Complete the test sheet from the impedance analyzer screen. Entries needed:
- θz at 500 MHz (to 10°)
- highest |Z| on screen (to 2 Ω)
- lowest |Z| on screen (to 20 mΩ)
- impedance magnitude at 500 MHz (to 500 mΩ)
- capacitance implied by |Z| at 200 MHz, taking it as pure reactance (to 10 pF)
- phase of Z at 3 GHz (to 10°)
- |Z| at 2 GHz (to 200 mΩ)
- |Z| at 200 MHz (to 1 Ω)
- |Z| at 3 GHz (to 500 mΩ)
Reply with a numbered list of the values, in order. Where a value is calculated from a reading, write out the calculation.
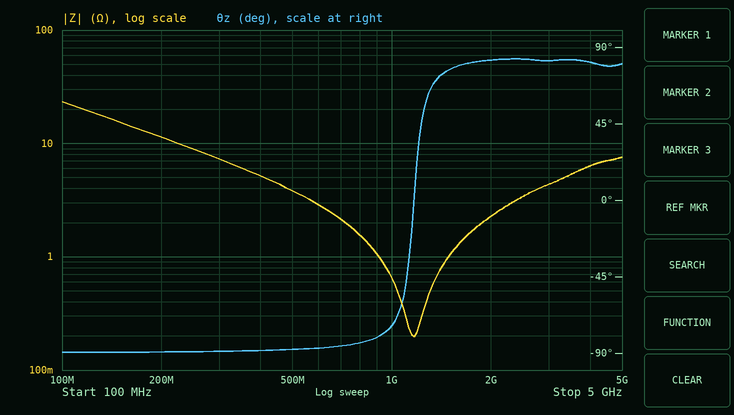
1. -90°
2. 24 Ω
3. 200 mΩ
4. 4.0 Ω
5. C = 1/(2π × 200 MHz × 11 Ω) ≈ 72.3 pF, so 70 pF to the nearest 10 pF
6. 80°
7. 2.2 Ω
8. 11 Ω
9. 4.5 Ω
